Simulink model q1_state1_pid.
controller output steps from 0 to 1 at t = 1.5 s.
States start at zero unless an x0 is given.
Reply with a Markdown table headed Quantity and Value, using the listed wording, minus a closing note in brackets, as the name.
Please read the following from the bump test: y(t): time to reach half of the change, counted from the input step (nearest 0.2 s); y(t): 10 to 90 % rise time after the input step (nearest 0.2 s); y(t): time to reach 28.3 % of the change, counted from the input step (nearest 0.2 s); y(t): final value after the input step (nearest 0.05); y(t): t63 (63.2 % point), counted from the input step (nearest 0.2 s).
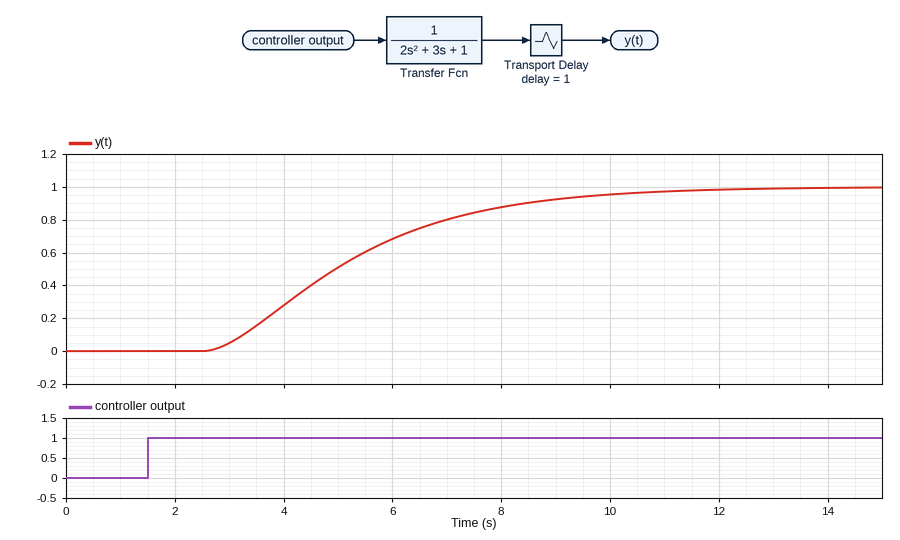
| Quantity | Value |
|---|---|
| y(t): time to reach half of the change, counted from the input step | 3.4 s |
| y(t): 10 to 90 % rise time after the input step | 5.2 s |
| y(t): time to reach 28.3 % of the change, counted from the input step | 2.6 s |
| y(t): final value after the input step | 1.00 |
| y(t): t63 (63.2 % point), counted from the input step | 4.2 s |
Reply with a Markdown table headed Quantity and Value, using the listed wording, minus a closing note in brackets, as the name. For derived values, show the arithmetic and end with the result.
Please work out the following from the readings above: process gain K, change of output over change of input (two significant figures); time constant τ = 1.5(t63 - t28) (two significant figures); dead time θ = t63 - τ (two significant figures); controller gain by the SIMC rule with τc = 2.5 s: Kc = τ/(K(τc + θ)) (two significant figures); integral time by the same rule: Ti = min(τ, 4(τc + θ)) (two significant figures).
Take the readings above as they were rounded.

| Quantity | Value |
|---|---|
| process gain K, change of output over change of input | (1 - 0) / 1 = 1.0 |
| time constant τ = 1.5(t63 - t28) | 1.5 × (4.2 - 2.6) = 2.4 s |
| dead time θ = t63 - τ | 4.2 - 2.4 = 1.8 s |
| controller gain by the SIMC rule with τc = 2.5 s: Kc = τ/(K(τc + θ)) | 2.4 / (1 × (2.5 + 1.8)) = 0.56 |
| integral time by the same rule: Ti = min(τ, 4(τc + θ)) | min(2.4, 4 × (2.5 + 1.8)) = 2.4 s |
